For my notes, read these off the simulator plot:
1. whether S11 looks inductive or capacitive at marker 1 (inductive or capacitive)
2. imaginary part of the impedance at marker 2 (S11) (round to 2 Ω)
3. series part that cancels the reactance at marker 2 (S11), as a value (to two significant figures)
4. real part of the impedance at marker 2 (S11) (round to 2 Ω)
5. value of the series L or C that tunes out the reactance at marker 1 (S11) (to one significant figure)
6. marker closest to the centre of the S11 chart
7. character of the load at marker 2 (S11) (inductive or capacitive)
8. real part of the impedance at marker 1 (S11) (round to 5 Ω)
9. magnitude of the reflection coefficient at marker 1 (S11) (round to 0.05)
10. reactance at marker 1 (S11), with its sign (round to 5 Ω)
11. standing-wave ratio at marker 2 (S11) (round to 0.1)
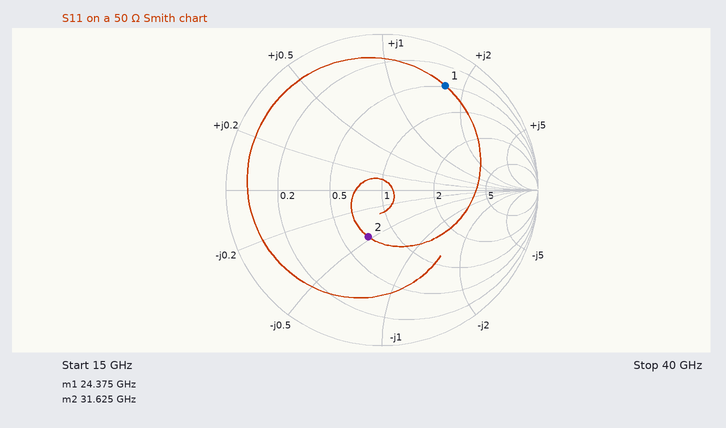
inductive
-24 Ω
120 pH
36 Ω
80 fF
marker 2
capacitive
25 Ω
0.80
+85 Ω
1.9
